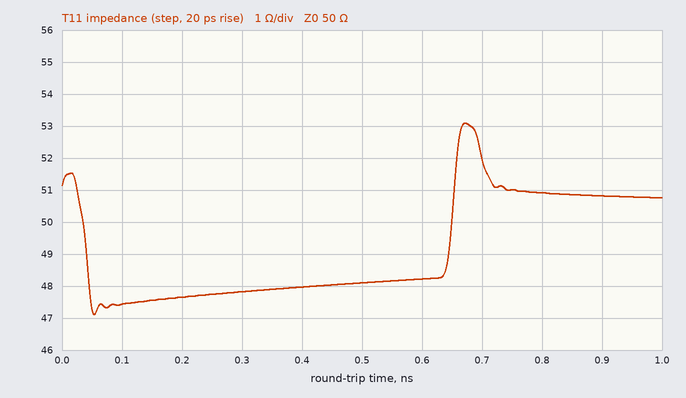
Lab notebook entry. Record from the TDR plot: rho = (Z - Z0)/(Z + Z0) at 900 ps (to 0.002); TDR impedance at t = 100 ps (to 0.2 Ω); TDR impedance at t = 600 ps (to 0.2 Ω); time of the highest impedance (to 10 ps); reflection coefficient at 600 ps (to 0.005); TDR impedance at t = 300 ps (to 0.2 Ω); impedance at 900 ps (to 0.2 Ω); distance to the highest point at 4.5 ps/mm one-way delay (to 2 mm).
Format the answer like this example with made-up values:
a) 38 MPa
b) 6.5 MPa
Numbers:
a) +0.008
b) 47.4 Ω
c) 48.2 Ω
d) 670 ps
e) -0.020
f) 47.8 Ω
g) 50.8 Ω
h) 74 mm
